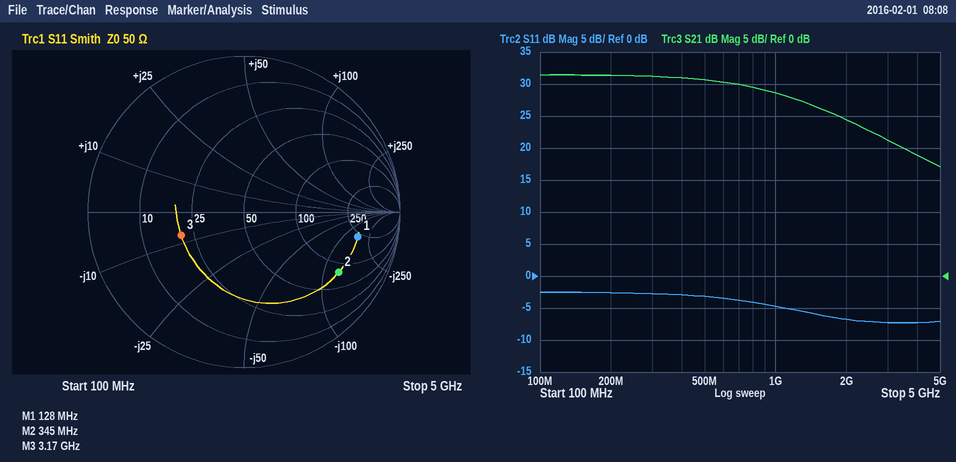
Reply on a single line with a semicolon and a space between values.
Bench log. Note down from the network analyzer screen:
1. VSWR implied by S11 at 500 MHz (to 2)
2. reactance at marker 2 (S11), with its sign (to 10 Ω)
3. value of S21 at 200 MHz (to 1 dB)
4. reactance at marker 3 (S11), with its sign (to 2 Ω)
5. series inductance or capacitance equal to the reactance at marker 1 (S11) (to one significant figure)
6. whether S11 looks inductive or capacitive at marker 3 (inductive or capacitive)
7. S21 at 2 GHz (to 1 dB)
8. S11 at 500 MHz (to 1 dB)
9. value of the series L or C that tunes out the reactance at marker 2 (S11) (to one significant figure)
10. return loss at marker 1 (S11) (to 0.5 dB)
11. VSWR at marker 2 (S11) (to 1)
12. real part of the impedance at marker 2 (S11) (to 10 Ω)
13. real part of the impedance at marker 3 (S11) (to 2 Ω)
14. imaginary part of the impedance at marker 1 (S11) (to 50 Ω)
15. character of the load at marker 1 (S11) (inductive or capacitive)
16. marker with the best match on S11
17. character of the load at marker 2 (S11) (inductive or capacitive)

6; -130 Ω; 31 dB; -8 Ω; 8 pF; capacitive; 24 dB; -3 dB; 60 nH; 2.5 dB; 6; 80 Ω; 20 Ω; -150 Ω; capacitive; marker 3; capacitive
